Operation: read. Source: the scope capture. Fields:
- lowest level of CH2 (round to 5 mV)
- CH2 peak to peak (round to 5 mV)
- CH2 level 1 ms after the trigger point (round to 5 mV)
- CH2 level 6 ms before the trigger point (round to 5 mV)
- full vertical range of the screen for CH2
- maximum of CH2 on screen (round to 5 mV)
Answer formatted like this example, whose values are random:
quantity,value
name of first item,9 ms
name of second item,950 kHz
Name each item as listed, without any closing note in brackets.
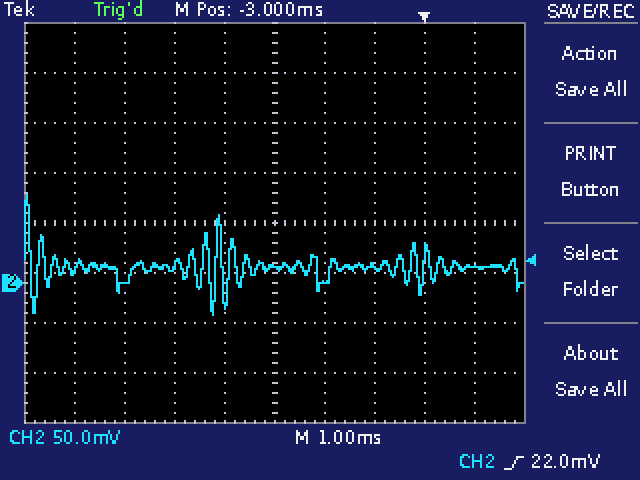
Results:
quantity,value
lowest level of CH2,-30 mV
CH2 peak to peak,120 mV
CH2 level 1 ms after the trigger point,15 mV
CH2 level 6 ms before the trigger point,0 mV
full vertical range of the screen for CH2,400 mV
maximum of CH2 on screen,90 mV
